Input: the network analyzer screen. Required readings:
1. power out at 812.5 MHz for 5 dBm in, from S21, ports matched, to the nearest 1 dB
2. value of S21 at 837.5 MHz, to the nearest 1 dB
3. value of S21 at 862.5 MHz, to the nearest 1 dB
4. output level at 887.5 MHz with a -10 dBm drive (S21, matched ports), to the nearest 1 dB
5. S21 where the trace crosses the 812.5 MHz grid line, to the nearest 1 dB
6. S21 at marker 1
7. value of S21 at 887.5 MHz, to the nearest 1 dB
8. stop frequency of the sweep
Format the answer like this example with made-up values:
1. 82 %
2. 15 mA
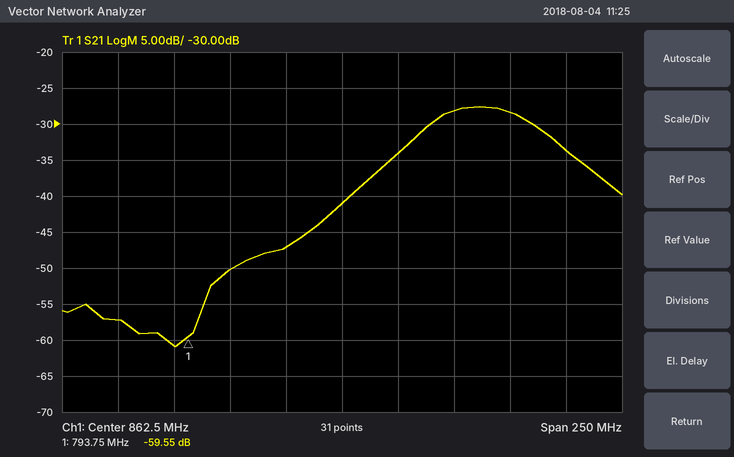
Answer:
1. -45 dBm
2. -47 dB
3. -41 dB
4. -44 dBm
5. -50 dB
6. -59.55 dB
7. -34 dB
8. 987.5 MHz
